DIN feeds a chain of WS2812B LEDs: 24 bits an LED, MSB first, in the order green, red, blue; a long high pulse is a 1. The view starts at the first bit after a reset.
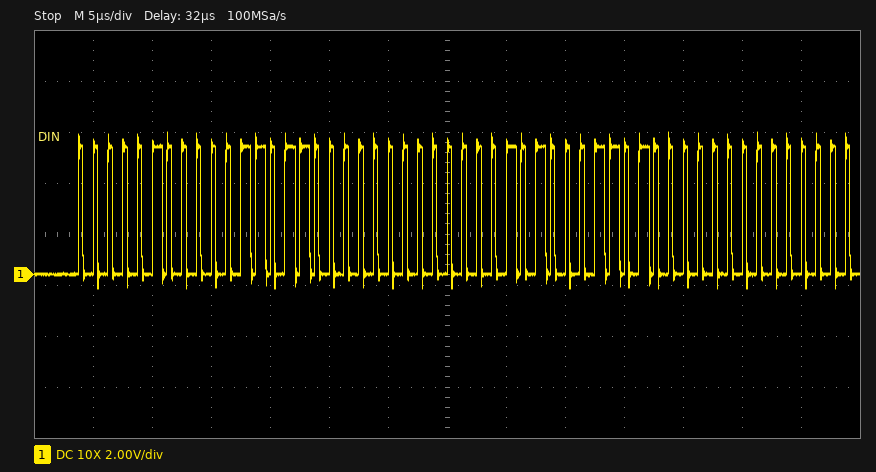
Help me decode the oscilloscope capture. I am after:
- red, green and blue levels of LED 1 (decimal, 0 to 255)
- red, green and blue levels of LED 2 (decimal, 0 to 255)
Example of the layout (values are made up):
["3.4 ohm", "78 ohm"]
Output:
["27, 4, 0", "26, 5, 0"]
